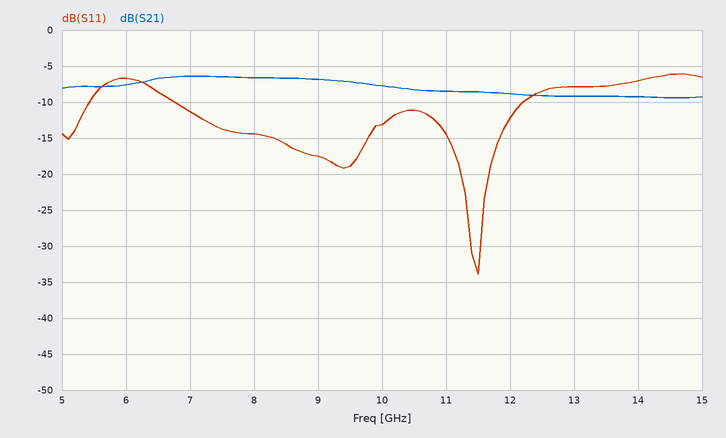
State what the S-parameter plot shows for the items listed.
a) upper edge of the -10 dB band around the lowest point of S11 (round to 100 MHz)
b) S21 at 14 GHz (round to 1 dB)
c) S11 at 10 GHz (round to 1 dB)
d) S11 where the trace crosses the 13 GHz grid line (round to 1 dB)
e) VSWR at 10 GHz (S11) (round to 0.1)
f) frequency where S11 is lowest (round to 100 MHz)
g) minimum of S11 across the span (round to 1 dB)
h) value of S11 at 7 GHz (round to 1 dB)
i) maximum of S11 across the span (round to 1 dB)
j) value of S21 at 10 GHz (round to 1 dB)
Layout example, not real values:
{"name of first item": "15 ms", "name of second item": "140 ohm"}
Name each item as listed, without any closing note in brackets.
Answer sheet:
{"upper edge of the -10 dB band around the lowest point of S11": "12.2 GHz", "S21 at 14 GHz": "-9 dB", "S11 at 10 GHz": "-13 dB", "S11 where the trace crosses the 13 GHz grid line": "-8 dB", "VSWR at 10 GHz (S11)": "1.6", "frequency where S11 is lowest": "11.5 GHz", "minimum of S11 across the span": "-34 dB", "value of S11 at 7 GHz": "-11 dB", "maximum of S11 across the span": "-6 dB", "value of S21 at 10 GHz": "-8 dB"}
